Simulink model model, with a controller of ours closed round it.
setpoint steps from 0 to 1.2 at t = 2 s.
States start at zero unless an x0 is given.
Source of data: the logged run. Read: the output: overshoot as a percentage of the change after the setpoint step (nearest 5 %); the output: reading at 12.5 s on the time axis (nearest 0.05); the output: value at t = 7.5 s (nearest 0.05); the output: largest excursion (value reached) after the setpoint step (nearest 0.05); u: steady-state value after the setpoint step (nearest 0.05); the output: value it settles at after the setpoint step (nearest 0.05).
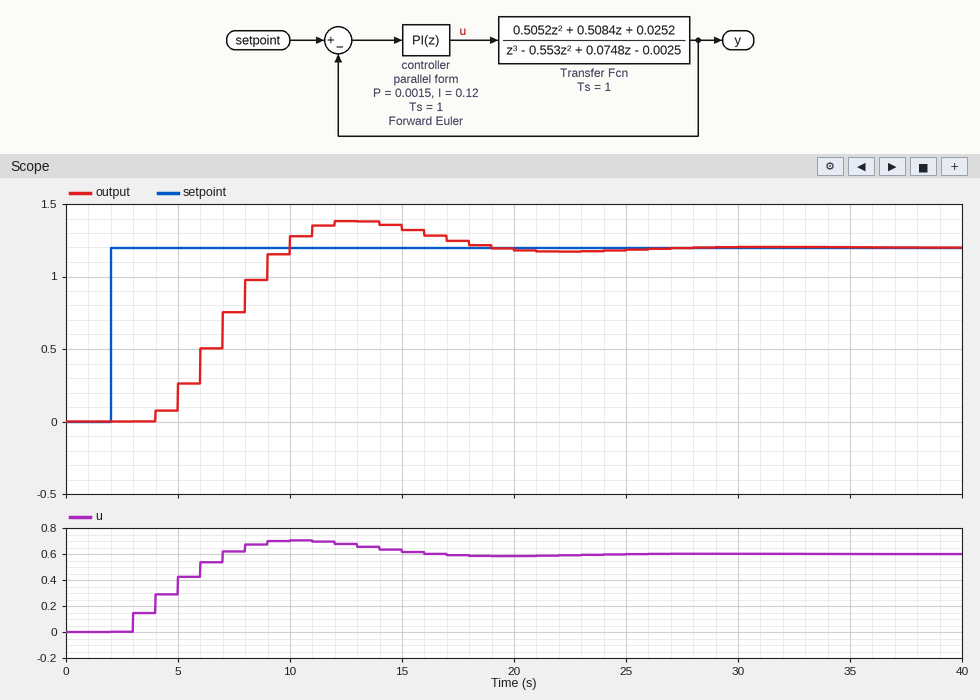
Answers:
15 %
1.40
0.75
1.40
0.60
1.20
